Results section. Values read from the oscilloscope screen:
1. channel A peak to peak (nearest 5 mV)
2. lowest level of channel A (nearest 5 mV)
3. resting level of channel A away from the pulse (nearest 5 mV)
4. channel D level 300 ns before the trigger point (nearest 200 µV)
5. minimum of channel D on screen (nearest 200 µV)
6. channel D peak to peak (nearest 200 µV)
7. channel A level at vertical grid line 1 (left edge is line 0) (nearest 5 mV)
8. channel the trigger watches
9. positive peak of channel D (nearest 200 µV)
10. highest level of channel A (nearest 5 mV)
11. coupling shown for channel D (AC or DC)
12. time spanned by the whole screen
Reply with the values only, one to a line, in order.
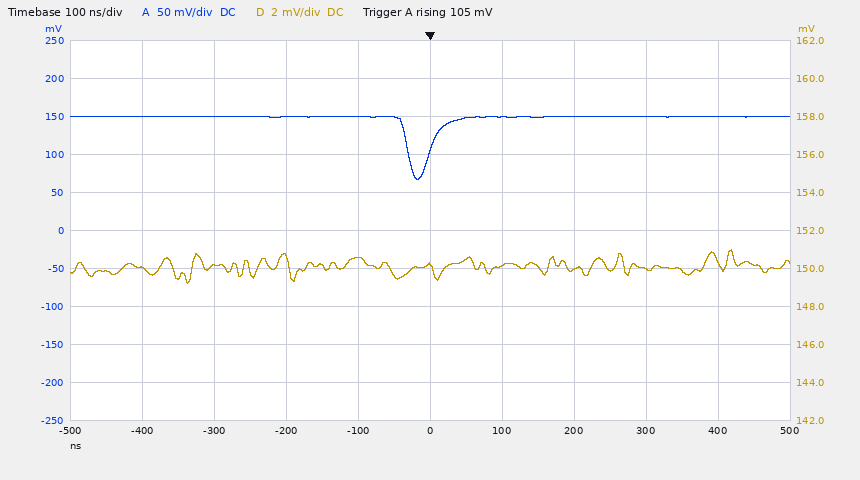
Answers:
85 mV
65 mV
150 mV
150.2 mV
149.2 mV
1.8 mV
150 mV
channel A
151.0 mV
150 mV
DC
1 µs
